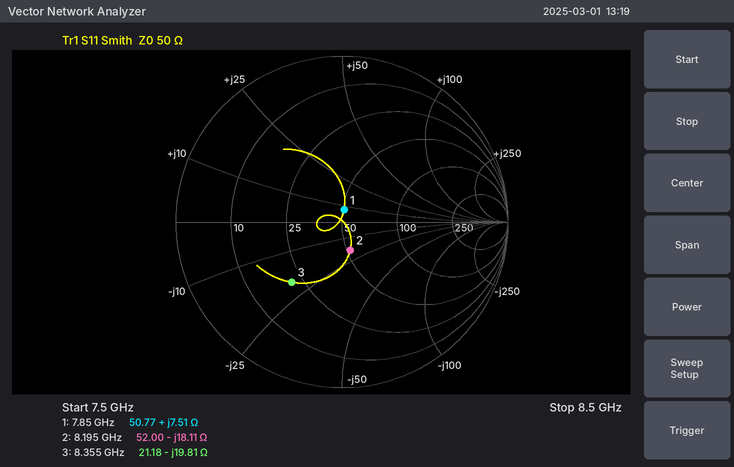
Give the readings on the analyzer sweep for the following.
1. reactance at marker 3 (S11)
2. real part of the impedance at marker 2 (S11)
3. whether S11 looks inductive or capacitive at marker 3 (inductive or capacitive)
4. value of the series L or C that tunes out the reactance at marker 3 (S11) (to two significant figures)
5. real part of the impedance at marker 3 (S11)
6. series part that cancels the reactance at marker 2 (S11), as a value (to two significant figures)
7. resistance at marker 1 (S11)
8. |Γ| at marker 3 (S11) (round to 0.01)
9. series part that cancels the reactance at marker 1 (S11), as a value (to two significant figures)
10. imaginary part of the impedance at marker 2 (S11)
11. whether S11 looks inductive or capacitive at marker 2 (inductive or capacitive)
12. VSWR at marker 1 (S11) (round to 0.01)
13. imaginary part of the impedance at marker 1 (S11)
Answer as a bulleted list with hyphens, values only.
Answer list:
- -19.81 Ω
- 52.00 Ω
- capacitive
- 380 pH
- 21.18 Ω
- 350 pH
- 50.77 Ω
- 0.47
- 2.7 pF
- -18.11 Ω
- capacitive
- 1.16
- +7.51 Ω
